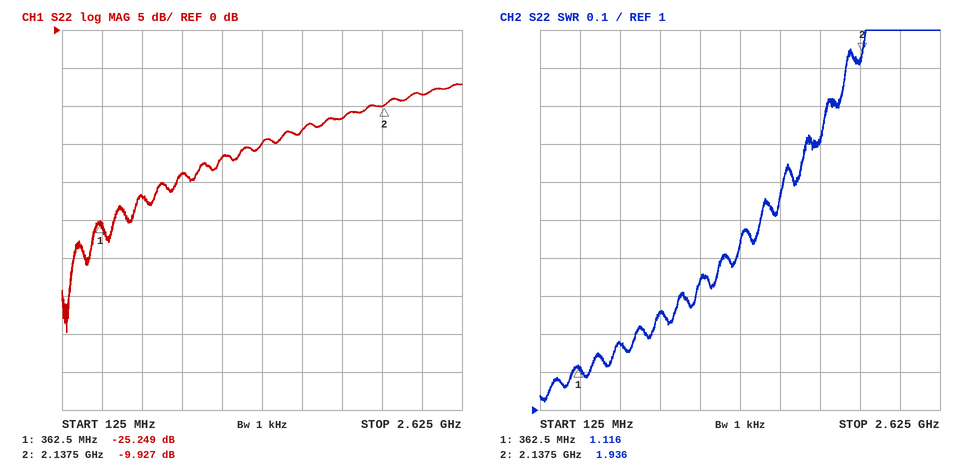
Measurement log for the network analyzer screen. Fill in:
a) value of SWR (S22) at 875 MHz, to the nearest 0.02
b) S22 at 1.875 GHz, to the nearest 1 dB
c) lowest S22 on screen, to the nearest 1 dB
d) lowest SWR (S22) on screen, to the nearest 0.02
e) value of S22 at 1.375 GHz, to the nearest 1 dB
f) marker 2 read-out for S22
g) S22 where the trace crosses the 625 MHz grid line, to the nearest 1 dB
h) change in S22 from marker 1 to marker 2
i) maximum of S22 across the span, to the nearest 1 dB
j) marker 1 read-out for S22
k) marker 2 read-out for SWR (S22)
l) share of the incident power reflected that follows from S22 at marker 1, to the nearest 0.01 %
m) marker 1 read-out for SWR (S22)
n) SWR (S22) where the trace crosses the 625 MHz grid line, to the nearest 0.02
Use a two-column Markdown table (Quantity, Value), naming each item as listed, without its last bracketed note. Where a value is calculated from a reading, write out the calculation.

| Quantity | Value |
|---|---|
| value of SWR (S22) at 875 MHz, to the nearest 0.02 | 1.26 |
| S22 at 1.875 GHz, to the nearest 1 dB | -12 dB |
| lowest S22 on screen, to the nearest 1 dB | -40 dB |
| lowest SWR (S22) on screen, to the nearest 0.02 | 1.02 |
| value of S22 at 1.375 GHz, to the nearest 1 dB | -15 dB |
| marker 2 read-out for S22 | -9.927 dB |
| S22 where the trace crosses the 625 MHz grid line, to the nearest 1 dB | -22 dB |
| change in S22 from marker 1 to marker 2 | -9.927 − (-25.249) = 15.322 dB |
| maximum of S22 across the span, to the nearest 1 dB | -7 dB |
| marker 1 read-out for S22 | -25.249 dB |
| marker 2 read-out for SWR | 1.936 |
| share of the incident power reflected that follows from S22 at marker 1, to the nearest 0.01 % | 10^(-25.249/10) ≈ 0.30 % |
| marker 1 read-out for SWR | 1.116 |
| SWR (S22) where the trace crosses the 625 MHz grid line, to the nearest 0.02 | 1.18 |
